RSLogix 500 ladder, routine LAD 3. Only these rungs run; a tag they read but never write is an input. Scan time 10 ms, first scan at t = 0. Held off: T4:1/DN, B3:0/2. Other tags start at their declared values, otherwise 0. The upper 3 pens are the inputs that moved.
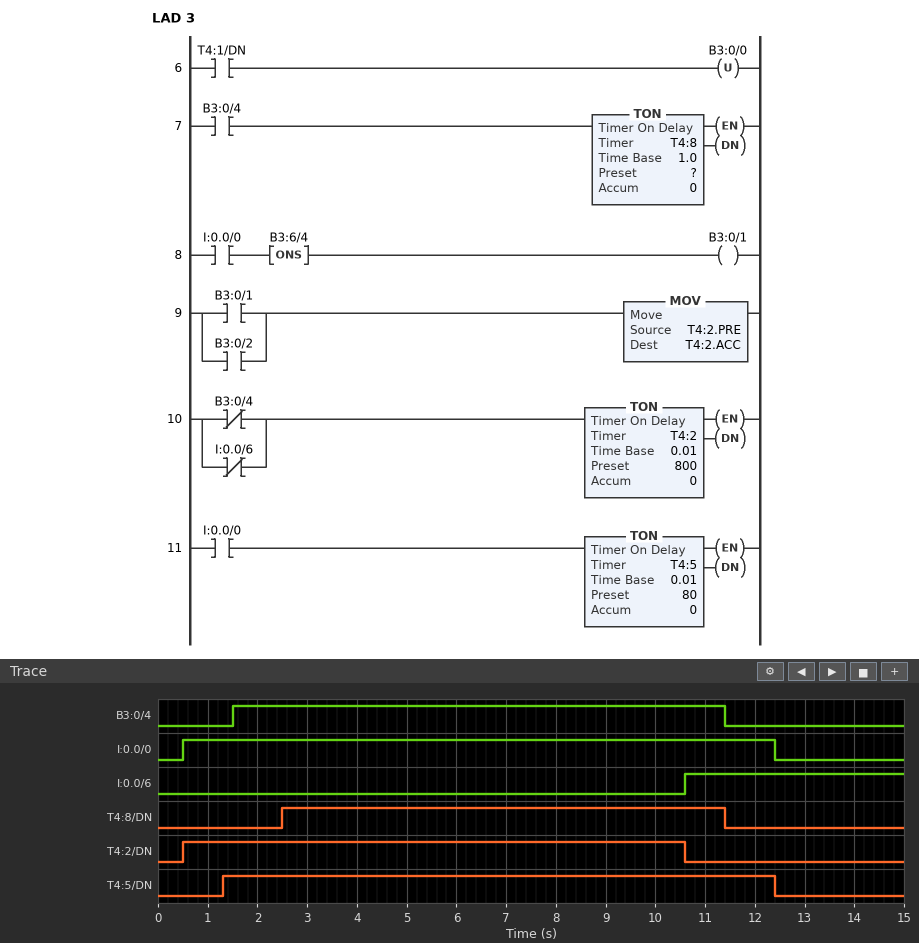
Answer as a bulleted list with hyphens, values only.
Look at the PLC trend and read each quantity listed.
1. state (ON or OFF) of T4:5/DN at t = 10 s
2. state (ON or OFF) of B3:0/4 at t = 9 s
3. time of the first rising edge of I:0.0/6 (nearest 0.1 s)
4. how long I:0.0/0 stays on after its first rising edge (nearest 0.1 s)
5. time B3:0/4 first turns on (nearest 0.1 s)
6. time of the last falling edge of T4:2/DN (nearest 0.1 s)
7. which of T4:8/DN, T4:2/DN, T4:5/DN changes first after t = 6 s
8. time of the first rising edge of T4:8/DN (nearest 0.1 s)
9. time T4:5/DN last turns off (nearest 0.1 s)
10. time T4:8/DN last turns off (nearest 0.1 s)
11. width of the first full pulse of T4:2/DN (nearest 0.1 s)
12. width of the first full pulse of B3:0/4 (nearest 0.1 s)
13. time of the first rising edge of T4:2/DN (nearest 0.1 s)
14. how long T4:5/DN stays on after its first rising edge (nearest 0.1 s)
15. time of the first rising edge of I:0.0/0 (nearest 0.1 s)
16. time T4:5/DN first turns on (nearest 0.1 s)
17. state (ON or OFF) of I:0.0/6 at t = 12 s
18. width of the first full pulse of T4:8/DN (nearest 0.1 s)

- ON
- ON
- 10.6 s
- 11.9 s
- 1.5 s
- 10.6 s
- T4:2/DN
- 2.5 s
- 12.4 s
- 11.4 s
- 10.1 s
- 9.9 s
- 0.5 s
- 11.1 s
- 0.5 s
- 1.3 s
- ON
- 8.9 s
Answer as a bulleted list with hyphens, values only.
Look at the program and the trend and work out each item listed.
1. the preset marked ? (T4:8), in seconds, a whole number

- 1 s
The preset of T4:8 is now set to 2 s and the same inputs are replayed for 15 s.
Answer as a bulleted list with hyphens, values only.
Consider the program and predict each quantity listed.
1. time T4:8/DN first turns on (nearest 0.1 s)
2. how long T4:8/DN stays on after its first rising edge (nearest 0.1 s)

- 3.5 s
- 7.9 s
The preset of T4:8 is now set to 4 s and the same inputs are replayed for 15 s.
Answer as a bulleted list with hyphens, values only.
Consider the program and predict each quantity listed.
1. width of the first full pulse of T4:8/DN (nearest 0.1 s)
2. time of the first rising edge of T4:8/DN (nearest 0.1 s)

- 5.9 s
- 5.5 s
